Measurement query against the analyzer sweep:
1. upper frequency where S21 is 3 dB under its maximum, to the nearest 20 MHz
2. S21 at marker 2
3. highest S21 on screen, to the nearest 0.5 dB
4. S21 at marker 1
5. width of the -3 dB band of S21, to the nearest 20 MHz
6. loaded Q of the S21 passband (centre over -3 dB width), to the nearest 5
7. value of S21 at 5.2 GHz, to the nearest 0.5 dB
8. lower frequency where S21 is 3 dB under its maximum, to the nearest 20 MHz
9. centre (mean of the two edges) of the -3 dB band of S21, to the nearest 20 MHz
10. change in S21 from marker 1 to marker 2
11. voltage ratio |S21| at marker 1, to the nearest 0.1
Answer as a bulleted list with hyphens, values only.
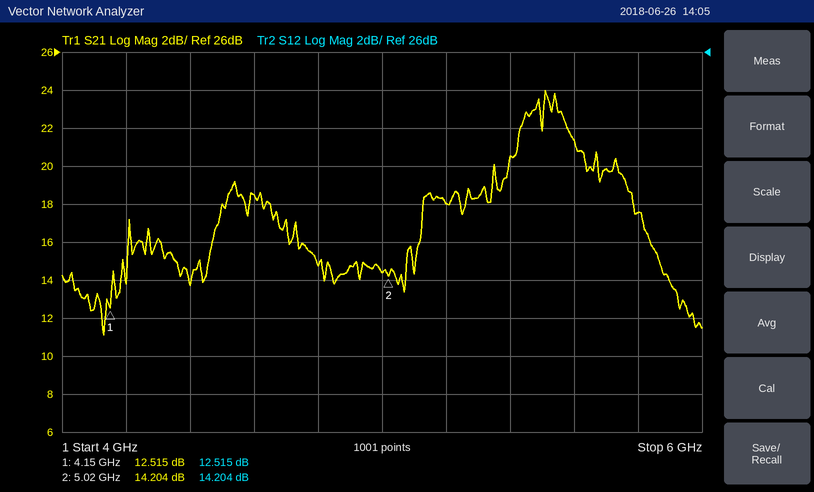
- 5.60 GHz
- 14.204 dB
- 24.0 dB
- 12.515 dB
- 180 MHz
- 30
- 18.0 dB
- 5.42 GHz
- 5.52 GHz
- 1.689 dB
- 4.2
